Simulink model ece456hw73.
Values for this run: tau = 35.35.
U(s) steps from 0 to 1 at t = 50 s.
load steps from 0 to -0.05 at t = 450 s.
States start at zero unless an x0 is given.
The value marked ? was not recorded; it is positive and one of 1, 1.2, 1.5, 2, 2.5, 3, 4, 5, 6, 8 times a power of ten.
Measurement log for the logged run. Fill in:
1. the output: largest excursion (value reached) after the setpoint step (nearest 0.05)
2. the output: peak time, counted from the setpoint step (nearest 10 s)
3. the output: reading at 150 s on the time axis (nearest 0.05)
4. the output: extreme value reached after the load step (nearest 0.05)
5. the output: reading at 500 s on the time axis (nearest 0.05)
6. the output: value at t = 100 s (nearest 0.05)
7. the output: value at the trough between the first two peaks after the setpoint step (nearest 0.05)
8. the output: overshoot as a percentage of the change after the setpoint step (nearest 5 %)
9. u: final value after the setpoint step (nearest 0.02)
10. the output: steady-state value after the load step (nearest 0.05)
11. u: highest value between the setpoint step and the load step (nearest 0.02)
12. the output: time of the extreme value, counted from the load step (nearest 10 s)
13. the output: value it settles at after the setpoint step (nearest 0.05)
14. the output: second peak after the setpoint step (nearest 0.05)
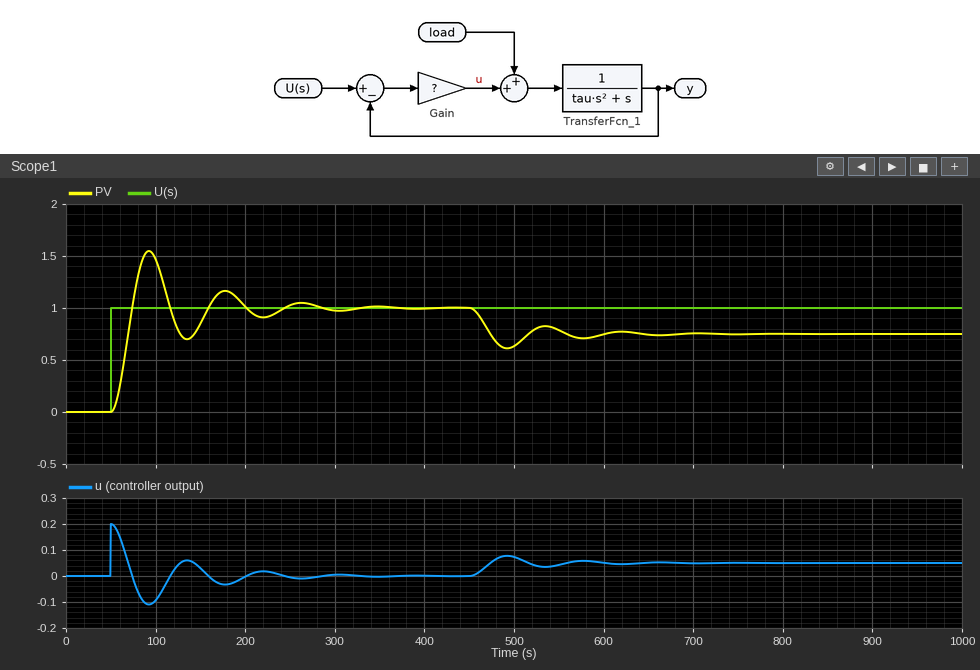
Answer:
1.55
40 s
0.85
0.60
0.65
1.45
0.70
55 %
0.00
0.75
0.20
40 s
1.00
1.15
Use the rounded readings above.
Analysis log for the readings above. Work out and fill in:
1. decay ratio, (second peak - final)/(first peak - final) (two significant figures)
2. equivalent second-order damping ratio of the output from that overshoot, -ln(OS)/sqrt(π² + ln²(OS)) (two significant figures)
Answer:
0.27
0.19
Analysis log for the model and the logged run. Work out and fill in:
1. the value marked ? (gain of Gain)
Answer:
0.2
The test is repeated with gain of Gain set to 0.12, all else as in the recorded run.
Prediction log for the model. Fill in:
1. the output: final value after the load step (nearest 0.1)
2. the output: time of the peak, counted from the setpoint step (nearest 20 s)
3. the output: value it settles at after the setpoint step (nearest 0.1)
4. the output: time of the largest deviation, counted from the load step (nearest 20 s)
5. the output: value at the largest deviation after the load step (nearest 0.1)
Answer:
0.6
60 s
1.0
60 s
0.4
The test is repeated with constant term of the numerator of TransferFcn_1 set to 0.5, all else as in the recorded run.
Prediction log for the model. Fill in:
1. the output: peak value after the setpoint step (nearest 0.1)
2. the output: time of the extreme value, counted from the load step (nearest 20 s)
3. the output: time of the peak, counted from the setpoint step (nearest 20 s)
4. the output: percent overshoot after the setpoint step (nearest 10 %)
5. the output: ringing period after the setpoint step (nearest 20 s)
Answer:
1.4
60 s
60 s
40 %
120 s
